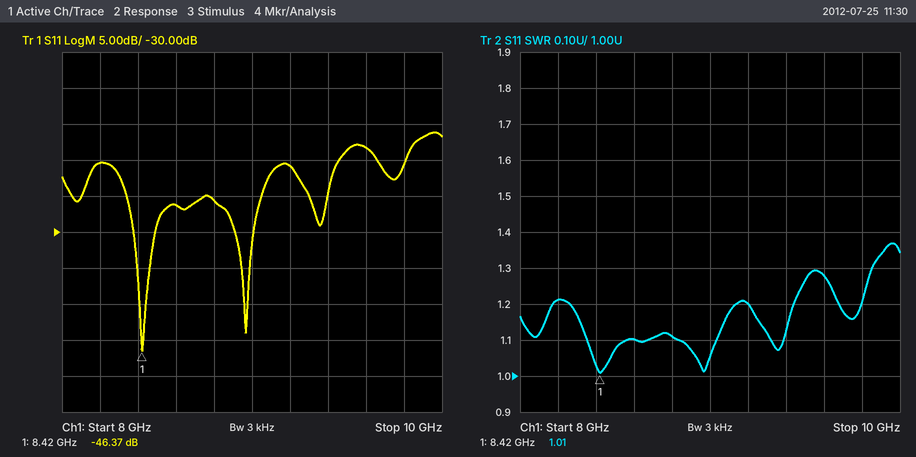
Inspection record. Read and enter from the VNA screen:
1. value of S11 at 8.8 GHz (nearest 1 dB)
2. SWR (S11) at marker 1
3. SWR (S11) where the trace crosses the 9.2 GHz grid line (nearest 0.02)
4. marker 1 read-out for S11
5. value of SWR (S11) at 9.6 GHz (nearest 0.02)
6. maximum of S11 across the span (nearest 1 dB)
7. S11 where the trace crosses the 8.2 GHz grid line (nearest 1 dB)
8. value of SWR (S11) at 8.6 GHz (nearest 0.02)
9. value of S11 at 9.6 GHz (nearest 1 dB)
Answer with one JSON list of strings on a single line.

["-26 dB", "1.01", "1.20", "-46.37 dB", "1.28", "-16 dB", "-20 dB", "1.10", "-18 dB"]
